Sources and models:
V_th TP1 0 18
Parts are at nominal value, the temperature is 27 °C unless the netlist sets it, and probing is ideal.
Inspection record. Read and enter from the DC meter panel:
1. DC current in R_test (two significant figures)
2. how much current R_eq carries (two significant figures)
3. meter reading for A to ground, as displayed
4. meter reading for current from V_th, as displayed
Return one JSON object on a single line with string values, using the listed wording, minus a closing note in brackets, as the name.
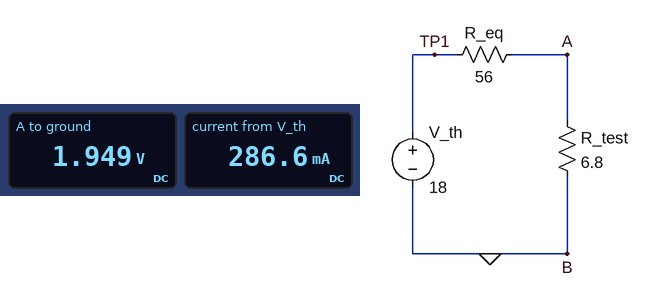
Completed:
{"DC current in R_test": "290 mA", "how much current R_eq carries": "290 mA", "meter reading for A to ground, as displayed": "1.949 V", "meter reading for current from V_th, as displayed": "286.6 mA"}
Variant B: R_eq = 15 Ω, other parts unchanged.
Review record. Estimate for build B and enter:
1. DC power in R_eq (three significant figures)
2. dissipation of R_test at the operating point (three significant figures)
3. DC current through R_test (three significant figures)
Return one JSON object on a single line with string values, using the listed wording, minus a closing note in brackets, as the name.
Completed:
{"DC power in R_eq": "10.2 W", "dissipation of R_test at the operating point": "4.64 W", "DC current through R_test": "826 mA"}
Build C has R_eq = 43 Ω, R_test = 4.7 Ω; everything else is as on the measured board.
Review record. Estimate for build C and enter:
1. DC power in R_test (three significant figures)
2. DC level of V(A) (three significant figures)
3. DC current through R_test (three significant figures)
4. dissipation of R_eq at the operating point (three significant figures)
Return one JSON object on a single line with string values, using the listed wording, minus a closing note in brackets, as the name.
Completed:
{"DC power in R_test": "669 mW", "DC level of V(A)": "1.77 V", "DC current through R_test": "377 mA", "dissipation of R_eq at the operating point": "6.12 W"}
